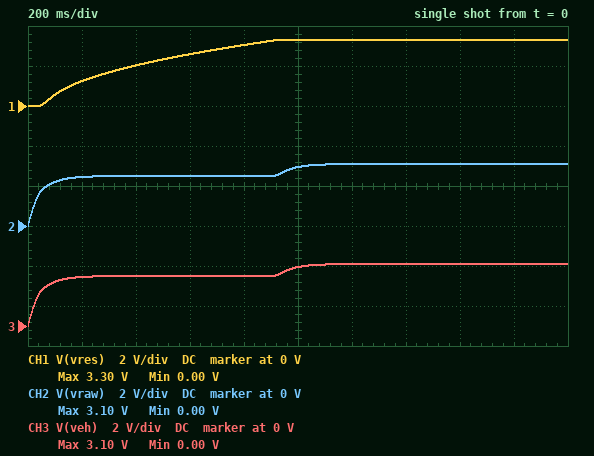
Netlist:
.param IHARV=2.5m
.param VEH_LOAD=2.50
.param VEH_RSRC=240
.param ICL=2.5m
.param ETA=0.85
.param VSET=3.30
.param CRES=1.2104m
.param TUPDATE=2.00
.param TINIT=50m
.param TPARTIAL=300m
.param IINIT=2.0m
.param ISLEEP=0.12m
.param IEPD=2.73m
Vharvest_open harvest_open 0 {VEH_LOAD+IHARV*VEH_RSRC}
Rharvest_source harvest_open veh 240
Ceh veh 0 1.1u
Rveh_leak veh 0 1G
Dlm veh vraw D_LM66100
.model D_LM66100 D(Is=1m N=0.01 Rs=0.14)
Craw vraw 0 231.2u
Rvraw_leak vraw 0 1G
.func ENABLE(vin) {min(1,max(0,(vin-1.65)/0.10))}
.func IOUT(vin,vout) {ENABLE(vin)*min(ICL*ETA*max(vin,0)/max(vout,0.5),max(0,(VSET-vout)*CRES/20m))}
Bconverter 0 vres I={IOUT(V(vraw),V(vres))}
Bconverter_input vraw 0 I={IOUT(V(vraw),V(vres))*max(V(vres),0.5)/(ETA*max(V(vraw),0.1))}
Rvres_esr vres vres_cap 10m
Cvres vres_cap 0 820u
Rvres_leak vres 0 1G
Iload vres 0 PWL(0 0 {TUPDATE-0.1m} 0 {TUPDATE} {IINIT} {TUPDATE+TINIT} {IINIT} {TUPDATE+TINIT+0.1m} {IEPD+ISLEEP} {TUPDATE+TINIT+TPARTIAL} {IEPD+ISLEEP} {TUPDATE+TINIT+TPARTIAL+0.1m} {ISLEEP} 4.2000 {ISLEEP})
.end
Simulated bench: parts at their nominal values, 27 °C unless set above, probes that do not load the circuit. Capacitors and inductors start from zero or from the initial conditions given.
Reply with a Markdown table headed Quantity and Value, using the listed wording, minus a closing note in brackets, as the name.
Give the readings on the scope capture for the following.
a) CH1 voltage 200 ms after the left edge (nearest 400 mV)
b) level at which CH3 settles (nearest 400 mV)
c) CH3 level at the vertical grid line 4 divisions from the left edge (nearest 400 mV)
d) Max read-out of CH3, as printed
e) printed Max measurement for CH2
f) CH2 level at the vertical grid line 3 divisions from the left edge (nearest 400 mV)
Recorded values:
| Quantity | Value |
|---|---|
| CH1 voltage 200 ms after the left edge | 1.2 V |
| level at which CH3 settles | 3.2 V |
| CH3 level at the vertical grid line 4 divisions from the left edge | 2.4 V |
| Max read-out of CH3, as printed | 3.10 V |
| printed Max measurement for CH2 | 3.10 V |
| CH2 level at the vertical grid line 3 divisions from the left edge | 2.4 V |
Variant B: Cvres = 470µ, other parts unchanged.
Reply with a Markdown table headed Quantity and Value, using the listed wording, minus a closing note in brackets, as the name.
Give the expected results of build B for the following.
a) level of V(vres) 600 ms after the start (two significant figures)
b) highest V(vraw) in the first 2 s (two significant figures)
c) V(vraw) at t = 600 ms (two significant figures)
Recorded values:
| Quantity | Value |
|---|---|
| level of V(vres) 600 ms after the start | 3.3 V |
| highest V(vraw) in the first 2 s | 3.1 V |
| V(vraw) at t = 600 ms | 2.8 V |
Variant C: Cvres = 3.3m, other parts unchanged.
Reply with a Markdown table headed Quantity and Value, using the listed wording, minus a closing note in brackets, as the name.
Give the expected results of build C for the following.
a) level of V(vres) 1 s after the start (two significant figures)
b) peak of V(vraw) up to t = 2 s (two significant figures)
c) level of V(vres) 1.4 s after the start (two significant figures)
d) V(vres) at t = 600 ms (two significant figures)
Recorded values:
| Quantity | Value |
|---|---|
| level of V(vres) 1 s after the start | 1.7 V |
| peak of V(vraw) up to t = 2 s | 2.5 V |
| level of V(vres) 1.4 s after the start | 2.0 V |
| V(vres) at t = 600 ms | 1.2 V |
